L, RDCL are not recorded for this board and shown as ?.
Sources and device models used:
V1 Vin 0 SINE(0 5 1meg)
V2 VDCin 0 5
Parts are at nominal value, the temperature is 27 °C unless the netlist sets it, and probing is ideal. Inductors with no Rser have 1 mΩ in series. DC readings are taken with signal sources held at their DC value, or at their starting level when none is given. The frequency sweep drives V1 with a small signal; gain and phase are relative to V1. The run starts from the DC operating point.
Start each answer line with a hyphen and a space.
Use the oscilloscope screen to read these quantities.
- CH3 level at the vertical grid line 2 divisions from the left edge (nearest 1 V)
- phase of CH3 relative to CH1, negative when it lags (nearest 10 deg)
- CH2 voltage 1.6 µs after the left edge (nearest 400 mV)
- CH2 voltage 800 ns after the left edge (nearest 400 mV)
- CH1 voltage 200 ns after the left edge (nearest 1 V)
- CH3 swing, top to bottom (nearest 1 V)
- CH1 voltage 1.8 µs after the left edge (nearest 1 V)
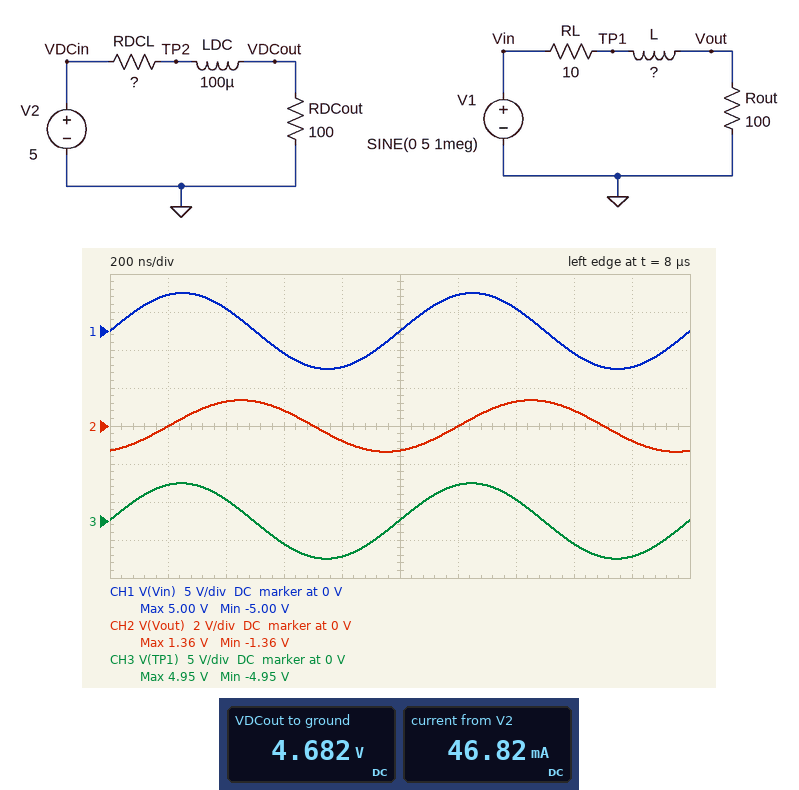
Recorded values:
- 3 V
- 0 deg
- 800 mV
- -800 mV
- 5 V
- 10 V
- -5 V
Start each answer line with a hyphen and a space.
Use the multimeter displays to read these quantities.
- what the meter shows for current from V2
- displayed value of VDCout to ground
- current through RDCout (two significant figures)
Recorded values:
- 46.82 mA
- 4.682 V
- 47 mA
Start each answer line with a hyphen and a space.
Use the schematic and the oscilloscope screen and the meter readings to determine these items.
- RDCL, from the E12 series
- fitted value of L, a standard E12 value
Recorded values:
- 6.8 Ω
- 56 µH
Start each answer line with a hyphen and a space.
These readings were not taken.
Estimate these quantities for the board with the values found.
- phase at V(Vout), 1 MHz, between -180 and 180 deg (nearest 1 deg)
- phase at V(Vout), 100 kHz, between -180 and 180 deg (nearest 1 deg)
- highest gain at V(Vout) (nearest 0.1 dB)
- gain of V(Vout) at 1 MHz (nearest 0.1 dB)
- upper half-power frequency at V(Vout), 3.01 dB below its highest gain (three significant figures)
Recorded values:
- -73 deg
- -18 deg
- -0.8 dB
- -11.3 dB
- 313 kHz
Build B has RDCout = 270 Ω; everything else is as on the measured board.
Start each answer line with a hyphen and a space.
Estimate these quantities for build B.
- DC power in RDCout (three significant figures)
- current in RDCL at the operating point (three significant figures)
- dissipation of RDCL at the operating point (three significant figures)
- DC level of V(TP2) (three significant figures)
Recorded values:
- 88.1 mW
- 18.1 mA
- 2.22 mW
- 4.88 V
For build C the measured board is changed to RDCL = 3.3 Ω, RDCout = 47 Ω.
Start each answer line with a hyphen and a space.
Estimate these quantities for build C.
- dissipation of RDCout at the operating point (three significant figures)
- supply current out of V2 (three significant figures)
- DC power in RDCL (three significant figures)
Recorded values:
- 464 mW
- 99.4 mA
- 32.6 mW
